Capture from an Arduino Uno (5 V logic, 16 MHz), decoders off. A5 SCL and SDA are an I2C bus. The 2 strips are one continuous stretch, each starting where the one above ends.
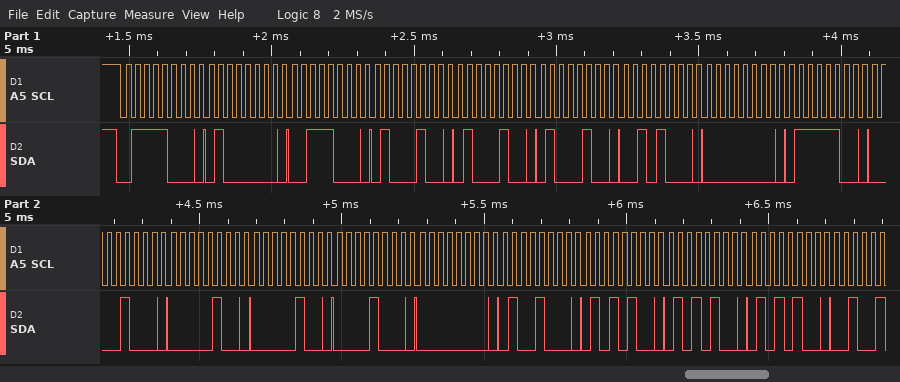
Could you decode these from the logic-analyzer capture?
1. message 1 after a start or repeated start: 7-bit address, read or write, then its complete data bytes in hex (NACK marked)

0x3C write: 40 38 44 44 44 28 00 7C 08 04 04 08 00 48 54 54 54
